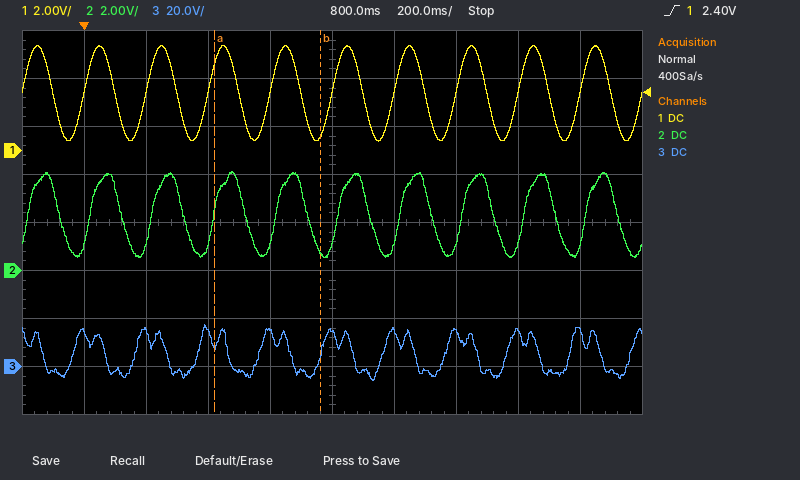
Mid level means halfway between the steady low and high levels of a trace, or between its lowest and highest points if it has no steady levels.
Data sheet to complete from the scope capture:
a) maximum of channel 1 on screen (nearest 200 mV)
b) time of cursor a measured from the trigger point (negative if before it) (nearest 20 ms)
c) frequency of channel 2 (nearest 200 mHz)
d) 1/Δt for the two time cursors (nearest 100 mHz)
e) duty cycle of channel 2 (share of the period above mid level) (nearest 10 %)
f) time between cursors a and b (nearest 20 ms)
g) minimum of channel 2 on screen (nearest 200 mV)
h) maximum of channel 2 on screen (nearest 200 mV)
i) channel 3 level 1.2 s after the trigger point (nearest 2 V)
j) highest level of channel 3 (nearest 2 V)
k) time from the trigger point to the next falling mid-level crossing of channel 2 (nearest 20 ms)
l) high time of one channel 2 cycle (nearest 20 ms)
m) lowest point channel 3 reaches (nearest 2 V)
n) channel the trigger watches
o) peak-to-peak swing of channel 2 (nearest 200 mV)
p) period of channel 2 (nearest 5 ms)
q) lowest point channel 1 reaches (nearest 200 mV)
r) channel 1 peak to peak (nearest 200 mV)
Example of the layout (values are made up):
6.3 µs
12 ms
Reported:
4.4 V
+420 ms
5.0 Hz
2.9 Hz
50 %
340 ms
600 mV
4.2 V
14 V
18 V
120 ms
100 ms
-6 V
channel 1
3.6 V
200 ms
400 mV
4.0 V
